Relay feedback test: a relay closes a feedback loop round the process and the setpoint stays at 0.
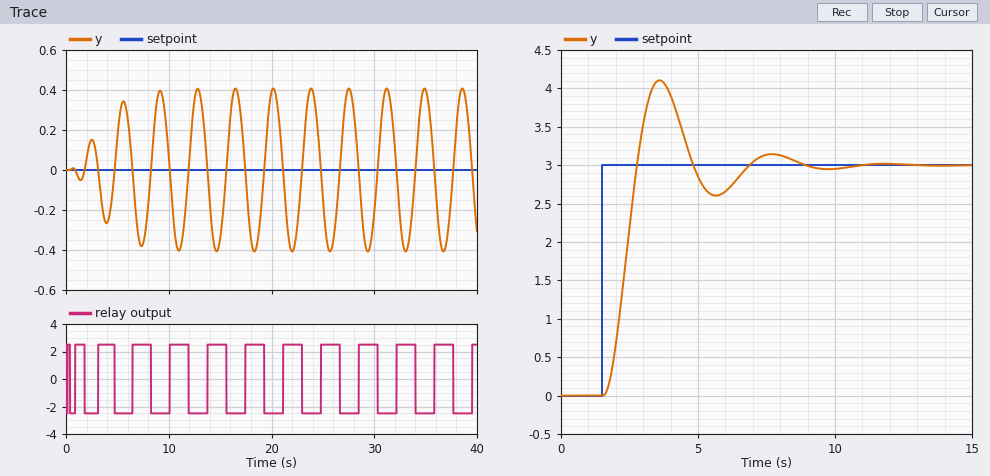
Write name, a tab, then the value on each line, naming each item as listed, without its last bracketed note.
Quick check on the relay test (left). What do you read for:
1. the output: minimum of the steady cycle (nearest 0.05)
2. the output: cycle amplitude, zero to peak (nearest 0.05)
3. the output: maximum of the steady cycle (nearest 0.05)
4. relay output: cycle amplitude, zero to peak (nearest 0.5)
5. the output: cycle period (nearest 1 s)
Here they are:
the output: minimum of the steady cycle	-0.40
the output: cycle amplitude, zero to peak	0.40
the output: maximum of the steady cycle	0.40
relay output: cycle amplitude, zero to peak	2.5
the output: cycle period	4 s
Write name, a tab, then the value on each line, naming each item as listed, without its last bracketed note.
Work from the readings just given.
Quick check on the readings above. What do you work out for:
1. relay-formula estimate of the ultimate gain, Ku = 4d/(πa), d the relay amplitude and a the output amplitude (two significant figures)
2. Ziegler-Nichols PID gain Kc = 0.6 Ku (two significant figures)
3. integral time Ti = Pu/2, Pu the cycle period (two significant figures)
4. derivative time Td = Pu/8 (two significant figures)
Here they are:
relay-formula estimate of the ultimate gain, Ku = 4d/(πa), d the relay amplitude and a the output amplitude	8.0
Ziegler-Nichols PID gain Kc = 0.6 Ku	4.8
integral time Ti = Pu/2, Pu the cycle period	2.0 s
derivative time Td = Pu/8	0.50 s
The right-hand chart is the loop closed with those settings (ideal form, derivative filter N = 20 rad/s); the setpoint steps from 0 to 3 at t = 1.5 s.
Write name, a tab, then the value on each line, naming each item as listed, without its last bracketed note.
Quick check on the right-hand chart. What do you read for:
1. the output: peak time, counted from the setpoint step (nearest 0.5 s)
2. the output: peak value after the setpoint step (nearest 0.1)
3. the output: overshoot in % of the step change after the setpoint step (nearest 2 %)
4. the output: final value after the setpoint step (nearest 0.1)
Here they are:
the output: peak time, counted from the setpoint step	2.0 s
the output: peak value after the setpoint step	4.1
the output: overshoot in % of the step change after the setpoint step	36 %
the output: final value after the setpoint step	3.0
